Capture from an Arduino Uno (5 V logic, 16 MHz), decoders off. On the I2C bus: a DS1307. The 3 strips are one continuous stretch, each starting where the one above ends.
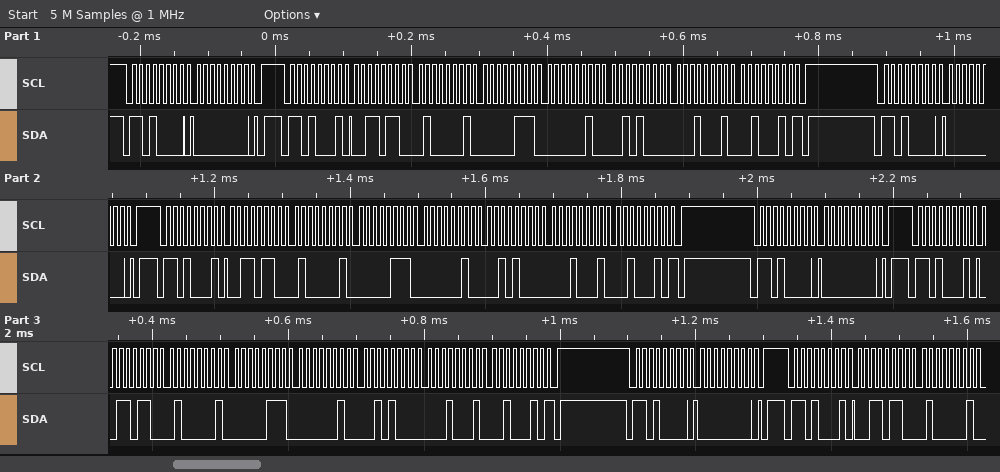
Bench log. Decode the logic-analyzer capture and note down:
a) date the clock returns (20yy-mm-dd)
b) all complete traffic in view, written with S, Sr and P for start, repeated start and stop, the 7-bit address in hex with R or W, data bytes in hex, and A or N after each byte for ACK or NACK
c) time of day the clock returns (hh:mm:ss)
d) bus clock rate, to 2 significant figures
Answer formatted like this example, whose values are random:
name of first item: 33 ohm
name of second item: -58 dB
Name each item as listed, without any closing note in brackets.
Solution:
date the clock returns: 2022-11-28
all complete traffic in view, written with S, Sr and P for start, repeated start and stop, the 7-bit address in hex with R or W, data bytes in hex, and A or N after each byte for ACK or NACK: S 68W A 00 A P S 68R A 36 A 41 A 07 A 02 A 28 A 11 A 22 N P S 68W A 00 A P S 68R A 36 A 41 A 07 A 02 A 28 A 11 A 22 N P S 68W A 00 A P S 68R A 36 A 41 A 07 A 02 A 28 A 11 A 22 N P S 68W A 00 A P S 68R A 36 A 41 A
time of day the clock returns: 07:41:36
bus clock rate, to 2 significant figures: 100 kHz
